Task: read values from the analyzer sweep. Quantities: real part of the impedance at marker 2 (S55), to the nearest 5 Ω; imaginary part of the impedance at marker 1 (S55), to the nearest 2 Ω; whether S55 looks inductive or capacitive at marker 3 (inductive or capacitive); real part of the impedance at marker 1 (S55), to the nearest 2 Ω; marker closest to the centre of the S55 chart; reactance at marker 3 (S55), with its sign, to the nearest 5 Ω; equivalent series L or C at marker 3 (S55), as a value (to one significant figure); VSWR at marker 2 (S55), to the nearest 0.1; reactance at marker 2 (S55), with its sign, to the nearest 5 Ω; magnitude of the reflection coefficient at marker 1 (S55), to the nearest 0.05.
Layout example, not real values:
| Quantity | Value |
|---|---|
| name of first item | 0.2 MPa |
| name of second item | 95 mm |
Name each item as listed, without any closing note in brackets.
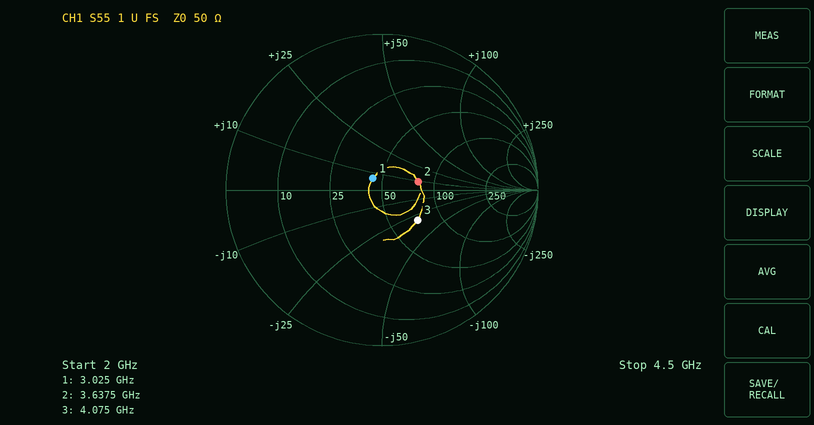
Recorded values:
| Quantity | Value |
|---|---|
| real part of the impedance at marker 2 (S55), to the nearest 5 Ω | 80 Ω |
| imaginary part of the impedance at marker 1 (S55), to the nearest 2 Ω | +6 Ω |
| whether S55 looks inductive or capacitive at marker 3 | capacitive |
| real part of the impedance at marker 1 (S55), to the nearest 2 Ω | 44 Ω |
| marker closest to the centre of the S55 chart | marker 1 |
| reactance at marker 3 (S55), with its sign, to the nearest 5 Ω | -30 Ω |
| equivalent series L or C at marker 3 (S55), as a value | 1 pF |
| VSWR at marker 2 (S55), to the nearest 0.1 | 1.6 |
| reactance at marker 2 (S55), with its sign, to the nearest 5 Ω | +10 Ω |
| magnitude of the reflection coefficient at marker 1 (S55), to the nearest 0.05 | 0.10 |
